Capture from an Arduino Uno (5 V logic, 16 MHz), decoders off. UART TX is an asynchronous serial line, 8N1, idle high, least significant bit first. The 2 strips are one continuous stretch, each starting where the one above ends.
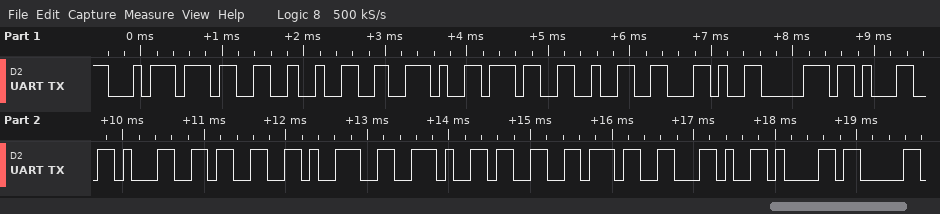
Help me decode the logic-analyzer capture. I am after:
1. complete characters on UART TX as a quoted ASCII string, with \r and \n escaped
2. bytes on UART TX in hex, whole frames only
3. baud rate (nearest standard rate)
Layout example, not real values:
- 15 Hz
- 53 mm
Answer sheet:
- "t32.72,p1139.37,a"
- 74 33 32 2E 37 32 2C 70 31 31 33 39 2E 33 37 2C 61
- 9600 baud
